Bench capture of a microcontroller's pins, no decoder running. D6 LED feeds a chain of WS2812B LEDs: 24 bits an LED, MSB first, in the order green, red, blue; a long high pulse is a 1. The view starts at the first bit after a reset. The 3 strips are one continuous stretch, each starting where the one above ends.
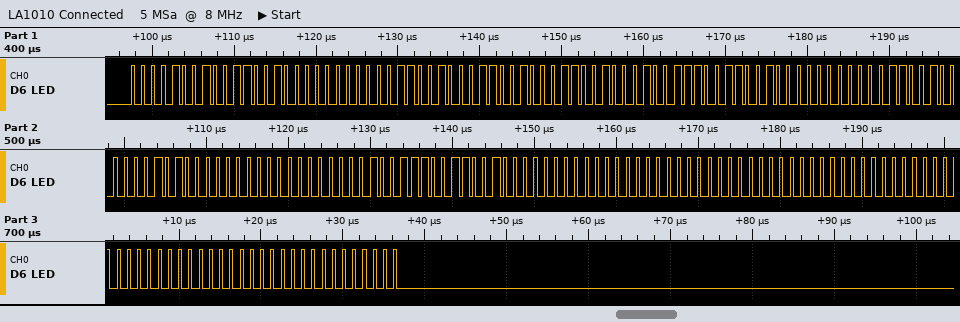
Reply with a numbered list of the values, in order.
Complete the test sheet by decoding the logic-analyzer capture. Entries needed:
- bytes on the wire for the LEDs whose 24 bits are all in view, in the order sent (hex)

1. 09 32 00 32 32 32 27 32 00 32 05 00 00 27 32 00 00 00 00 00 00 00 00 00
